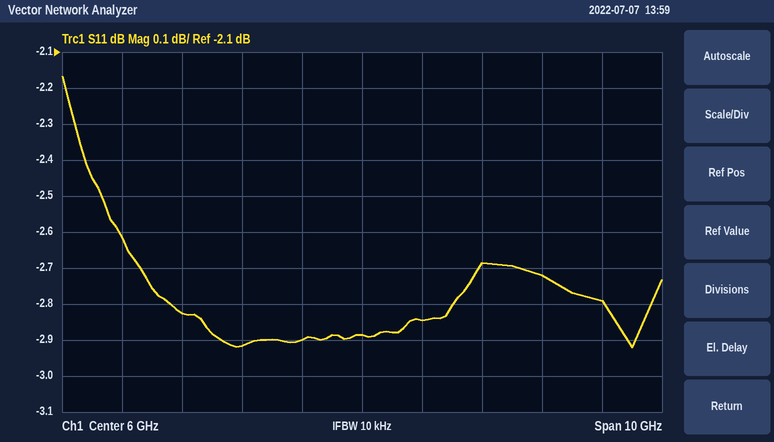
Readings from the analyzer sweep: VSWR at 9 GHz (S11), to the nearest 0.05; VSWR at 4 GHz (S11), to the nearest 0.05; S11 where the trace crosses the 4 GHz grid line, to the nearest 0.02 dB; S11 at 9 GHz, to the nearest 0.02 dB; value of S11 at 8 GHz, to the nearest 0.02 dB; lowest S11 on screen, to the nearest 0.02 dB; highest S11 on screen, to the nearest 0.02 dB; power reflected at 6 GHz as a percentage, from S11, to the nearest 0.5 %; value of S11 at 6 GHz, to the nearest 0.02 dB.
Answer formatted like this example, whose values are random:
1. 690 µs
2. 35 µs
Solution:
1. 6.45
2. 6.00
3. -2.92 dB
4. -2.72 dB
5. -2.68 dB
6. -2.92 dB
7. -2.16 dB
8. 51.5 %
9. -2.88 dB
